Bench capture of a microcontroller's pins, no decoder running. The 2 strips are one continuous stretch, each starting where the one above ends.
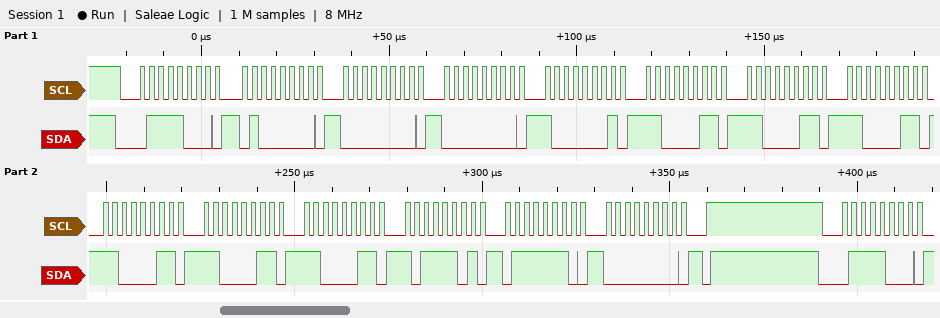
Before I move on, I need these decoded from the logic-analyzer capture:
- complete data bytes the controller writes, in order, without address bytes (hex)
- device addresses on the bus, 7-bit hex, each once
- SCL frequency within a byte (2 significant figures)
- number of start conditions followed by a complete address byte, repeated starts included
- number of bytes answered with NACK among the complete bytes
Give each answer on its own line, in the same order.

40 00 00 81 C3 C3 C3 C3 C3 C3 BD 7E 00
0x3C
400 kHz
2
0
